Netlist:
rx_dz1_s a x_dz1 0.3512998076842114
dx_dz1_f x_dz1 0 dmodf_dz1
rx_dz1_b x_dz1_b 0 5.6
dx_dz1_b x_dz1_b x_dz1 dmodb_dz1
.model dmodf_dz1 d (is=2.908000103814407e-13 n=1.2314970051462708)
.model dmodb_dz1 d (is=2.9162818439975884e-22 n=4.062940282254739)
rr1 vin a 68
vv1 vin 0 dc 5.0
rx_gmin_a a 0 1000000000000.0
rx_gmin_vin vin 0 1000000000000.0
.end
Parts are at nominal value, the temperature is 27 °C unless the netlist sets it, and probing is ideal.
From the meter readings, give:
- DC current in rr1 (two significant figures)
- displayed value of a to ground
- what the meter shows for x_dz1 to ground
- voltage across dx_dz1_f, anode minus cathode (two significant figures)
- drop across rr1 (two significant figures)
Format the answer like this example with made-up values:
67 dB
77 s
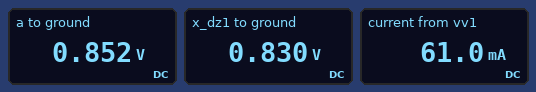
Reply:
61 mA
0.852 V
0.830 V
830 mV
4.1 V
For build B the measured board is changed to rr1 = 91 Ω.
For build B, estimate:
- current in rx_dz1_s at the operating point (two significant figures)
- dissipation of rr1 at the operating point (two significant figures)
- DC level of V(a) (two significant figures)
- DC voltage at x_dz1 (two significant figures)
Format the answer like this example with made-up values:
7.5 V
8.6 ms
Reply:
46 mA
190 mW
840 mV
820 mV
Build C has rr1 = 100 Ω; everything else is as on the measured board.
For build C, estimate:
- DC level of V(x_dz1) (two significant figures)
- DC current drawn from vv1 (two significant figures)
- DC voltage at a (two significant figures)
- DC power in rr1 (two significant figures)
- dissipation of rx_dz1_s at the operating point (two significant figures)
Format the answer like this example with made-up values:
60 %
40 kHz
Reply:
820 mV
42 mA
830 mV
170 mW
610 µW
